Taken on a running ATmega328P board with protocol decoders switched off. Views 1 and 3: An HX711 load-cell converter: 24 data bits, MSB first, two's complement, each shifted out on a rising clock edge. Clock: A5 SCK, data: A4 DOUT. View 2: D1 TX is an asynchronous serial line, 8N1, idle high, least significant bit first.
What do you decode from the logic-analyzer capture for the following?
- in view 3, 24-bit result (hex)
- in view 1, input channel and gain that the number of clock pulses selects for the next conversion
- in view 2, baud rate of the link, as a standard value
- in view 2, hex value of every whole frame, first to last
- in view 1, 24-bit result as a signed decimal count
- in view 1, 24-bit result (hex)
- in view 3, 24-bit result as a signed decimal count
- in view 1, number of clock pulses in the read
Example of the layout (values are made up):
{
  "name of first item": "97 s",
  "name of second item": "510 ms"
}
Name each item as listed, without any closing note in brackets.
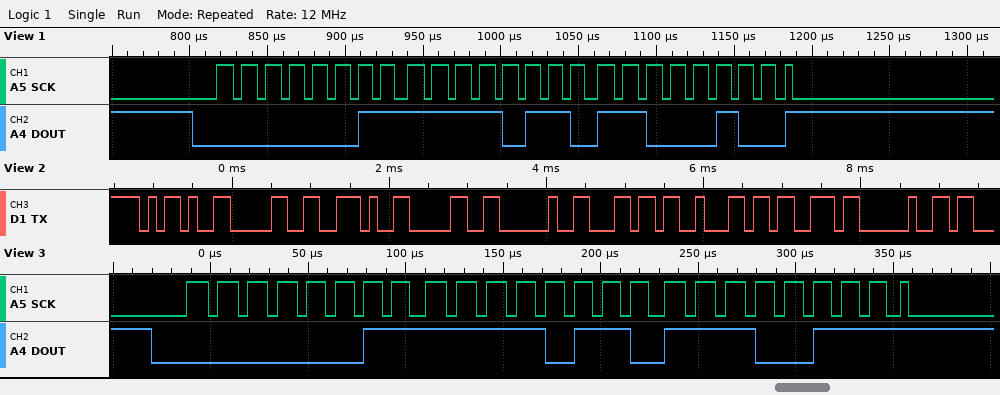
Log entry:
{
  "in view 3, 24-bit result": "0x03F6E7",
  "in view 1, input channel and gain that the number of clock pulses selects for the next conversion": "channel A, gain 128",
  "in view 2, baud rate of the link, as a standard value": "9600 baud",
  "in view 2, hex value of every whole frame, first to last": "2D 30 2E 30 20 6C 62 73 20",
  "in view 1, 24-bit result as a signed decimal count": "259780",
  "in view 1, 24-bit result": "0x03F6C4",
  "in view 3, 24-bit result as a signed decimal count": "259815",
  "in view 1, number of clock pulses in the read": "25"
}
